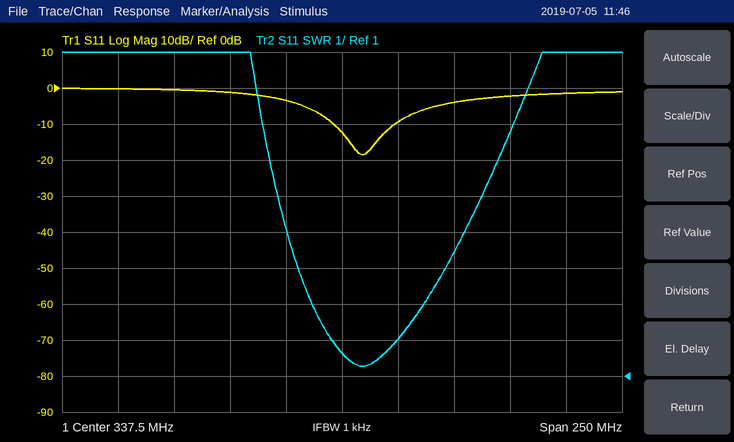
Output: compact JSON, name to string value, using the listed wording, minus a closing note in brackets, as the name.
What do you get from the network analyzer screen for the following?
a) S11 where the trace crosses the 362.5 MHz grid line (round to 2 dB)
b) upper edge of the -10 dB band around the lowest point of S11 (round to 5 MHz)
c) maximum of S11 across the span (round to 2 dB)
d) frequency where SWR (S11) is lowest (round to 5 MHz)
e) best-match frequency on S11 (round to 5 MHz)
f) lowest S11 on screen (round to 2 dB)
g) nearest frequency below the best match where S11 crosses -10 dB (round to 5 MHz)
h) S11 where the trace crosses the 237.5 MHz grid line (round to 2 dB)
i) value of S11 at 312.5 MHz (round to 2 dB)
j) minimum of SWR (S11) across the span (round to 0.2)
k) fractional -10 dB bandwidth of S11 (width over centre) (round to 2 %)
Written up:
{"S11 where the trace crosses the 362.5 MHz grid line": "-10 dB", "upper edge of the -10 dB band around the lowest point of S11": "360 MHz", "maximum of S11 across the span": "0 dB", "frequency where SWR (S11) is lowest": "345 MHz", "best-match frequency on S11": "345 MHz", "lowest S11 on screen": "-18 dB", "nearest frequency below the best match where S11 crosses -10 dB": "335 MHz", "S11 where the trace crosses the 237.5 MHz grid line": "0 dB", "value of S11 at 312.5 MHz": "-4 dB", "minimum of SWR (S11) across the span": "1.2", "fractional -10 dB bandwidth of S11 (width over centre)": "8 %"}
